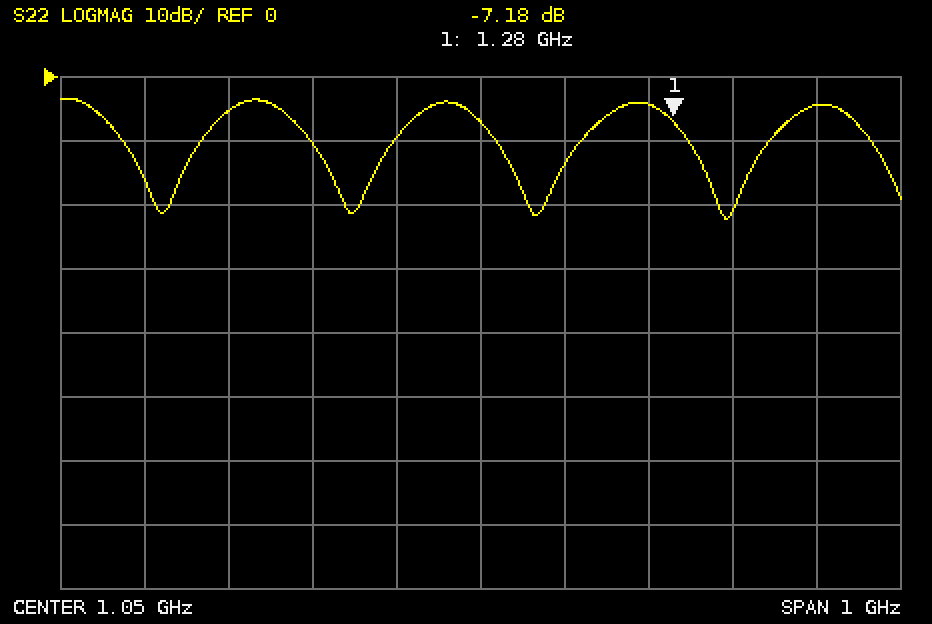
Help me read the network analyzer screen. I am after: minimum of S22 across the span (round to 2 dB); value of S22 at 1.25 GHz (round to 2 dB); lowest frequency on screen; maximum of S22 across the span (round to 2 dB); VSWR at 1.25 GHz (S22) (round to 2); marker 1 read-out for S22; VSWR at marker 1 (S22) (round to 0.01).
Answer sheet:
-22 dB
-4 dB
550 MHz
-4 dB
4
-7.18 dB
2.56
